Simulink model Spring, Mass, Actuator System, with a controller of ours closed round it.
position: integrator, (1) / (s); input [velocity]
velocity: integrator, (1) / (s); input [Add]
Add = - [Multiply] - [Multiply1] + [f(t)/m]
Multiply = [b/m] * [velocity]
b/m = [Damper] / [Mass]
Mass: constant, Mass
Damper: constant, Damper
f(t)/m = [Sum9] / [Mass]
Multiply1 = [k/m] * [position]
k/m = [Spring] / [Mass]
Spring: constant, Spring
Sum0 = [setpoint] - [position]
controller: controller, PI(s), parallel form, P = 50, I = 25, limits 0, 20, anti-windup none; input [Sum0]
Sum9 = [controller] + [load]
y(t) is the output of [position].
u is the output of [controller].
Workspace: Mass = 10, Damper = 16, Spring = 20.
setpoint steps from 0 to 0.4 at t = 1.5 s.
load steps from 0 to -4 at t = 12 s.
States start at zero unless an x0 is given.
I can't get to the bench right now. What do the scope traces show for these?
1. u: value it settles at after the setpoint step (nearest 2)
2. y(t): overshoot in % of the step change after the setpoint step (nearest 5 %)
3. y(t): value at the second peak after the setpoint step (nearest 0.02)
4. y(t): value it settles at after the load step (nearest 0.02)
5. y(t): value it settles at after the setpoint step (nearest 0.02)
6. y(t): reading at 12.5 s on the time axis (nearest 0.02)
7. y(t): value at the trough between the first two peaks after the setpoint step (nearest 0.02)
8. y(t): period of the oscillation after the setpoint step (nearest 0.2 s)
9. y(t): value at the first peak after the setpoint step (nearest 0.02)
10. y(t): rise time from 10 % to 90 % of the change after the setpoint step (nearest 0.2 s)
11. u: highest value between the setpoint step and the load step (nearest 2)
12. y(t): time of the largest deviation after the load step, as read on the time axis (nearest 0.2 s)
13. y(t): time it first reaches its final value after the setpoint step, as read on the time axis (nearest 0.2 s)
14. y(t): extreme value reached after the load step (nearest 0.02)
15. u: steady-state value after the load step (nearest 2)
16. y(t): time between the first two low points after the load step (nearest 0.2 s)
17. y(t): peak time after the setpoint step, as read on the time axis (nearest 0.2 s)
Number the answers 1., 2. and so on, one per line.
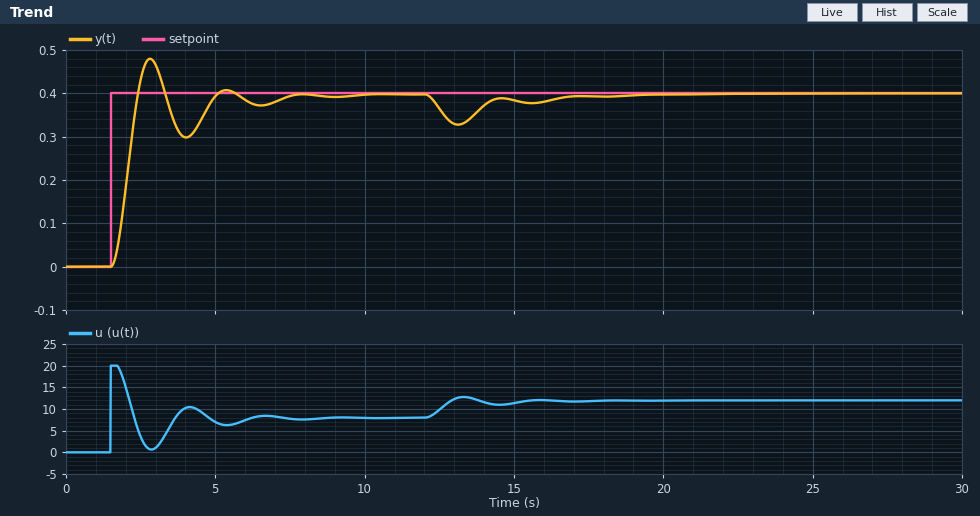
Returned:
1. 8
2. 20 %
3. 0.40
4. 0.40
5. 0.40
6. 0.36
7. 0.30
8. 2.6 s
9. 0.48
10. 0.6 s
11. 20
12. 13.2 s
13. 2.4 s
14. 0.32
15. 12
16. 2.4 s
17. 2.8 s
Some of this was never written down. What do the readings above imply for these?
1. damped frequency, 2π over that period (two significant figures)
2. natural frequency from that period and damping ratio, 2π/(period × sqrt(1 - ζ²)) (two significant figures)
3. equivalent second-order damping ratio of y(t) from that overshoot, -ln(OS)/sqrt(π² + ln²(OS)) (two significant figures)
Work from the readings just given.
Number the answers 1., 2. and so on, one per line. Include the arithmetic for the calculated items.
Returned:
1. 2π / 2.6 = 2.4 rad/s
2. 2π / (2.6 × sqrt(1 - 0.46²)) = 2.7 rad/s
3. ln(0.2) = -1.609; 1.609 / sqrt(9.870 + 2.590) = 0.46
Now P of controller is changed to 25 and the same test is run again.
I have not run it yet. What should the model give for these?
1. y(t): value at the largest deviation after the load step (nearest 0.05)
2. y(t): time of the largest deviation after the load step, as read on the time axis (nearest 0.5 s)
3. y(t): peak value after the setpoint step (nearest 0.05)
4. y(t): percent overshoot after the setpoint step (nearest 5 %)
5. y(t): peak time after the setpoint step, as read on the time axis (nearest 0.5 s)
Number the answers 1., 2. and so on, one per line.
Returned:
1. 0.30
2. 13.5 s
3. 0.45
4. 15 %
5. 3.5 s
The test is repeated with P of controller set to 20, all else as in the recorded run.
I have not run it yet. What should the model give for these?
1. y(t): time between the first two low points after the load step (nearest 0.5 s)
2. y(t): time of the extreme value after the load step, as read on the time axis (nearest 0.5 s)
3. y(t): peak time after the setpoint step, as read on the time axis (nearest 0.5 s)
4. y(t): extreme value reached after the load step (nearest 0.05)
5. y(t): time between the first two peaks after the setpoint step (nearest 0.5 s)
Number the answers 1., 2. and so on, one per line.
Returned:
1. 3.5 s
2. 13.5 s
3. 3.5 s
4. 0.30
5. 3.5 s
